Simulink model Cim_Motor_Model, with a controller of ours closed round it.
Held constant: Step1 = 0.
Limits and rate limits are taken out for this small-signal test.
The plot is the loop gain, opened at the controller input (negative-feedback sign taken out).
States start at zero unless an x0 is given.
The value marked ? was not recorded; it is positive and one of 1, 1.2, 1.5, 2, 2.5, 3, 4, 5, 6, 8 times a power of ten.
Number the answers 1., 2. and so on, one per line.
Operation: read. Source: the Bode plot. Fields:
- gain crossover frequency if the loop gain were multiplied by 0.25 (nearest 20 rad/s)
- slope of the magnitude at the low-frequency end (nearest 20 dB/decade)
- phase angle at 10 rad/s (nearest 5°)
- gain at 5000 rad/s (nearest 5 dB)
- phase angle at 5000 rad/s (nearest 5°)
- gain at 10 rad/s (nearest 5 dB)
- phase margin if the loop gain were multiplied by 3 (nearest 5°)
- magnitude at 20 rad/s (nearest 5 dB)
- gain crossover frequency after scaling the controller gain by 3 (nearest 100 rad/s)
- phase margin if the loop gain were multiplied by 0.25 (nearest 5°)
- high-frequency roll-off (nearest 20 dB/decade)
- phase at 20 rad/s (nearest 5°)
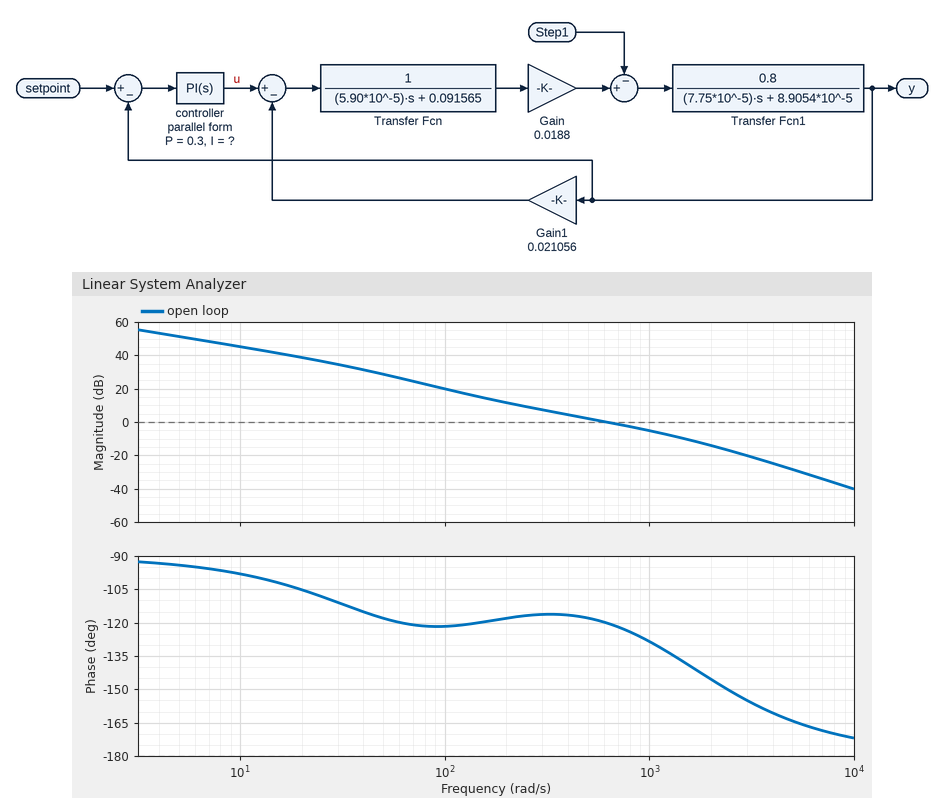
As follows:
1. 200 rad/s
2. -20 dB/decade
3. -100°
4. -30 dB
5. -165°
6. 45 dB
7. 45°
8. 40 dB
9. 1400 rad/s
10. 60°
11. -40 dB/decade
12. -105°
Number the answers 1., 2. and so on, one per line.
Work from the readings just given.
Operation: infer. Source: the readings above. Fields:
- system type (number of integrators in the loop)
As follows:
1. 1
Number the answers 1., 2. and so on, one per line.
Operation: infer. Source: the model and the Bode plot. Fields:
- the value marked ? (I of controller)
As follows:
1. 40
